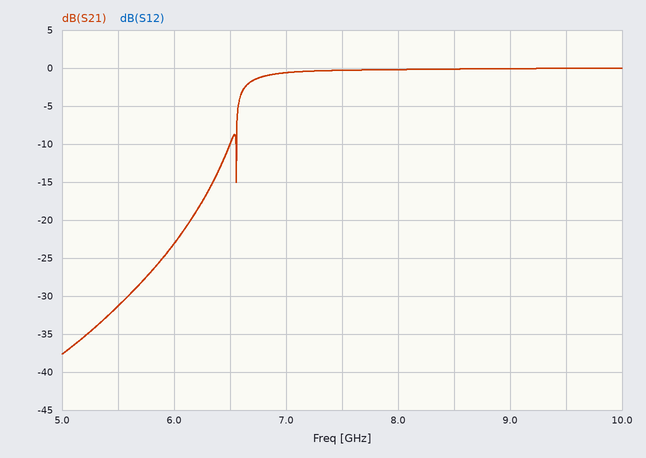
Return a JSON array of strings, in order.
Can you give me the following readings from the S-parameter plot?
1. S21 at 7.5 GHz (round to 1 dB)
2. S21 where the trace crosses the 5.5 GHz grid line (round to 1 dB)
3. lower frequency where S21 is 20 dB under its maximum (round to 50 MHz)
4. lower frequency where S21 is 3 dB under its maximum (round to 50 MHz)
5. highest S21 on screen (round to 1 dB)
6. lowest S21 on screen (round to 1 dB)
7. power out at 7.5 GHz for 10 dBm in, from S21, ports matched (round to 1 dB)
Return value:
["0 dB", "-31 dB", "6.15 GHz", "6.60 GHz", "0 dB", "-38 dB", "10 dBm"]
